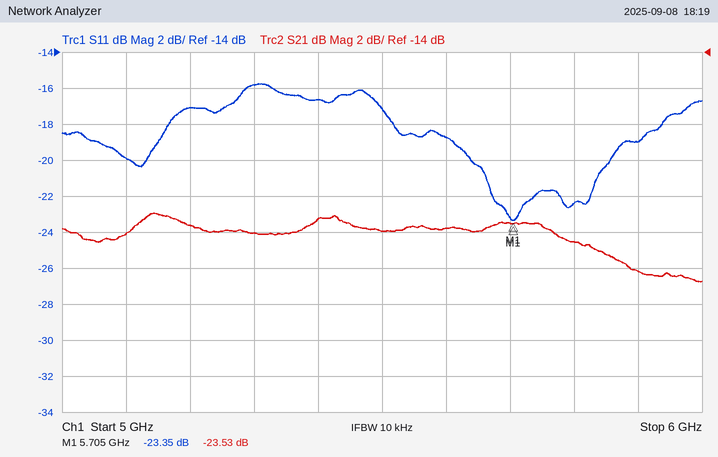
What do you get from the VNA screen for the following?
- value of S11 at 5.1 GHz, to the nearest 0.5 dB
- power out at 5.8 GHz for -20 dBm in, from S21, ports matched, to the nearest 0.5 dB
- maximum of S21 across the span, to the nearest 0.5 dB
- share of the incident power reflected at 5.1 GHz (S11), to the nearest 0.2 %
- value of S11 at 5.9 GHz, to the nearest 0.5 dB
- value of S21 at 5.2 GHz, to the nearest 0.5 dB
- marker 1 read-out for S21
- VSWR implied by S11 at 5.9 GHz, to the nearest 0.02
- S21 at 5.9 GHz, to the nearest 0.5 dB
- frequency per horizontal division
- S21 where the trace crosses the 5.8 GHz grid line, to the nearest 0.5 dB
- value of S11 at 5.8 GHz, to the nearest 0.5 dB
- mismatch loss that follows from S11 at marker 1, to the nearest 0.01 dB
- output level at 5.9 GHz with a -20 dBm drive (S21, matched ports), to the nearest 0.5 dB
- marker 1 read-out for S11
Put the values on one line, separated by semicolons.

-20.0 dB; -44.5 dBm; -23.0 dB; 1.0 %; -19.0 dB; -23.5 dB; -23.53 dB; 1.26; -26.0 dB; 100 MHz; -24.5 dB; -22.5 dB; 0.02 dB; -46.0 dBm; -23.35 dB
